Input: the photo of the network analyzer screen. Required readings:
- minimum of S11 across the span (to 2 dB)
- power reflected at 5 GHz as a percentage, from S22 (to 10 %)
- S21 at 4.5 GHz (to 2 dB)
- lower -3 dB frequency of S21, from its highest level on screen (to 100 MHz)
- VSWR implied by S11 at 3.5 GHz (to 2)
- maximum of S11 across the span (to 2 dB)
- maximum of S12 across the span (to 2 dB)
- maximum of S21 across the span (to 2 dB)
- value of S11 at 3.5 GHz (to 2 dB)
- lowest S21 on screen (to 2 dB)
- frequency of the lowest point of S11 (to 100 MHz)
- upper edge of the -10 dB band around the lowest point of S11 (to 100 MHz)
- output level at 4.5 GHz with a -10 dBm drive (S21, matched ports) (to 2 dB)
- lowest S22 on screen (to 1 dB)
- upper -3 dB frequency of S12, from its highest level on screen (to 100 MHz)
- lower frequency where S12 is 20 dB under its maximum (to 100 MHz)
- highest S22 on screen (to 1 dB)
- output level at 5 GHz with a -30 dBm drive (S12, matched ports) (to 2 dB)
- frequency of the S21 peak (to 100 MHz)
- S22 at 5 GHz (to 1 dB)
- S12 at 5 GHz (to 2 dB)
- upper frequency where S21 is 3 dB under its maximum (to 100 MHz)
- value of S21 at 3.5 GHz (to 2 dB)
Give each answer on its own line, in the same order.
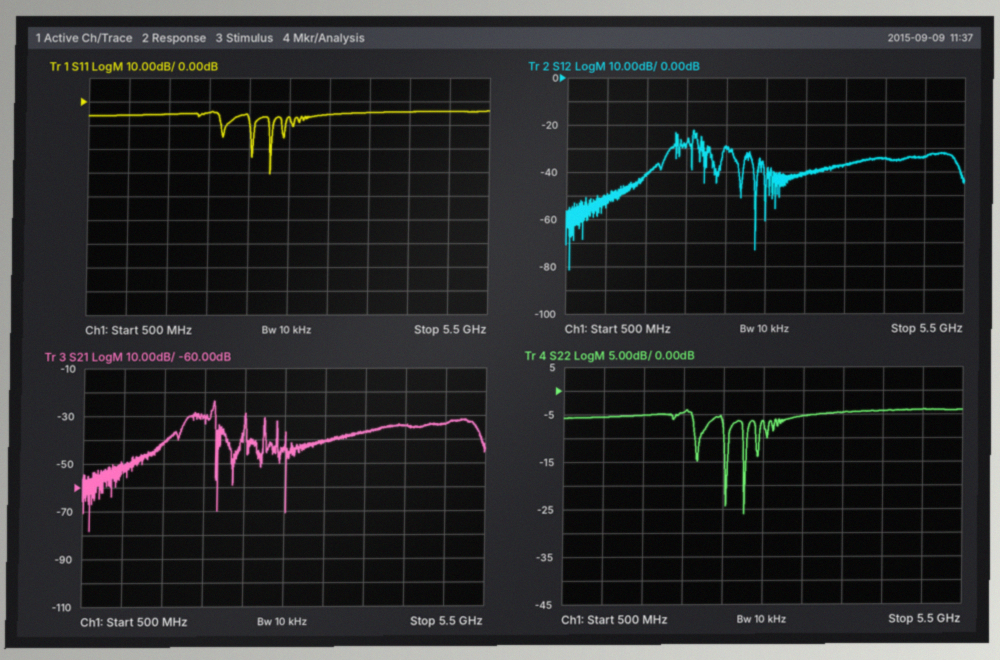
-30 dB
40 %
-34 dB
2.1 GHz
4
-4 dB
-22 dB
-24 dB
-6 dB
-78 dB
2.8 GHz
2.8 GHz
-44 dBm
-26 dB
2.1 GHz
1.5 GHz
-4 dB
-64 dBm
2.1 GHz
-4 dB
-34 dB
2.1 GHz
-40 dB
